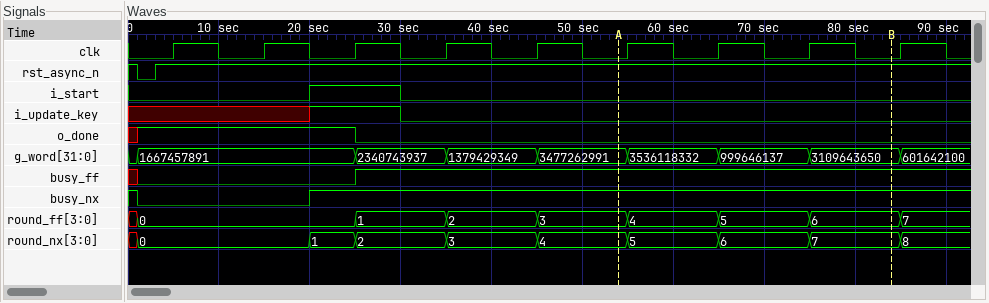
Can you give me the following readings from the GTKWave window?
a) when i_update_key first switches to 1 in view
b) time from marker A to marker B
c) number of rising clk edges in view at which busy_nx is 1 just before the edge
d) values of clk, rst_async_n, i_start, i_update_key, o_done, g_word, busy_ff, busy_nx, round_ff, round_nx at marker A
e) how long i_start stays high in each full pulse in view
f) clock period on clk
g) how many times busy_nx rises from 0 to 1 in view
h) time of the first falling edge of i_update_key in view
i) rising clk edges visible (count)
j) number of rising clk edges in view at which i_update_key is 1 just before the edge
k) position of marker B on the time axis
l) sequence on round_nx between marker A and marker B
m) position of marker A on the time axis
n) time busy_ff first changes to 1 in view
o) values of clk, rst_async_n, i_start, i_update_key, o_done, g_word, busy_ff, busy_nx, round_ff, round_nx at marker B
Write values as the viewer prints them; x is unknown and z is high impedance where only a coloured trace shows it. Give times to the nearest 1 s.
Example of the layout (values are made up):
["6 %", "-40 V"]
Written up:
["20 s", "30 s", "7", "clk=0, rst_async_n=1, i_start=0, i_update_key=0, o_done=0, g_word=3477262991, busy_ff=1, busy_nx=1, round_ff=3, round_nx=4", "10 s", "10 s", "1", "30 s", "9", "1", "84 s", "4, 5, 6, 7", "54 s", "25 s", "clk=0, rst_async_n=1, i_start=0, i_update_key=0, o_done=0, g_word=3109643650, busy_ff=1, busy_nx=1, round_ff=6, round_nx=7"]
